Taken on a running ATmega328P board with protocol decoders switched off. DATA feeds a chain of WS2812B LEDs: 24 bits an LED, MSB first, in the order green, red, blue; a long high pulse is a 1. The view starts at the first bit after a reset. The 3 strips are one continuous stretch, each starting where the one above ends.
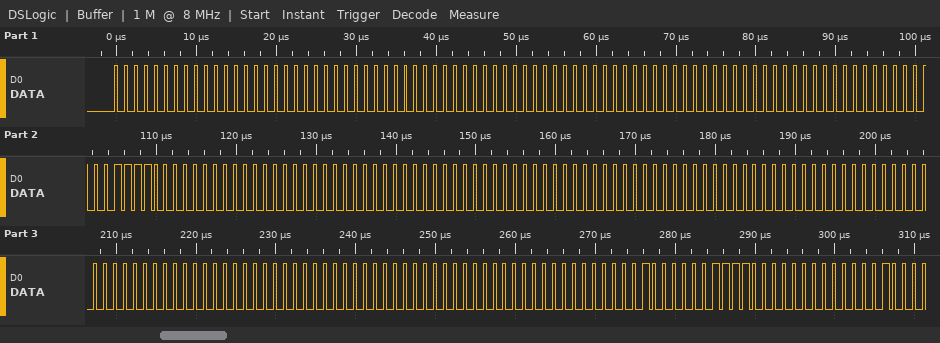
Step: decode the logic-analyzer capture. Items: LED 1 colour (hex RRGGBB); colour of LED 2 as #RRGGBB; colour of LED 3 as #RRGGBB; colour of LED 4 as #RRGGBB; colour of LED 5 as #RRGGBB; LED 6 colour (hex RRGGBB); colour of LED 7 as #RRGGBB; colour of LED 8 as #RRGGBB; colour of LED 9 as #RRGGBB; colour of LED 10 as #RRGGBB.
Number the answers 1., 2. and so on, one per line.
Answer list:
1. #000000
2. #000000
3. #000000
4. #0F0000
5. #000000
6. #000000
7. #000000
8. #000000
9. #000000
10. #0F0400
